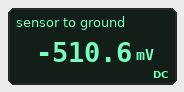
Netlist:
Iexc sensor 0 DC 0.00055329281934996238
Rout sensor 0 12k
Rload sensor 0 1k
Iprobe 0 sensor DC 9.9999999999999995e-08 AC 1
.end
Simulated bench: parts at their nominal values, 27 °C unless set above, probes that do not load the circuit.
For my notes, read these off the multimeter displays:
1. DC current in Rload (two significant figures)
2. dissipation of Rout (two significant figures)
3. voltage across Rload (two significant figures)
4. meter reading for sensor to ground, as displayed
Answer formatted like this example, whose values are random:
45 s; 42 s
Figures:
510 µA; 22 µW; 510 mV; -510.6 mV
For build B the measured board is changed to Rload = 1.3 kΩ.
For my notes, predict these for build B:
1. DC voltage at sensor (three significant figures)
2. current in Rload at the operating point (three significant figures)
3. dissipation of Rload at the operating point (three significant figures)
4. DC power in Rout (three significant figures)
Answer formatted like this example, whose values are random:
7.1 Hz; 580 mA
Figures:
-649 mV; 499 µA; 324 µW; 35.1 µW
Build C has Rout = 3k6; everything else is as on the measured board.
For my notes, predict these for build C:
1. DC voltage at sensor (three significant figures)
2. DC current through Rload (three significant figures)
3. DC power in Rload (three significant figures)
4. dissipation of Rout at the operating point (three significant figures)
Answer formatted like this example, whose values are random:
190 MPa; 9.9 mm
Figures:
-433 mV; 433 µA; 187 µW; 52.1 µW
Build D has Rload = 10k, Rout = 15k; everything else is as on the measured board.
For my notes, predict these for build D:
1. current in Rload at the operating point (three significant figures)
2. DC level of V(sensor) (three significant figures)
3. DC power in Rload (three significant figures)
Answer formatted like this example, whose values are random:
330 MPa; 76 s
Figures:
332 µA; -3.32 V; 1.10 mW
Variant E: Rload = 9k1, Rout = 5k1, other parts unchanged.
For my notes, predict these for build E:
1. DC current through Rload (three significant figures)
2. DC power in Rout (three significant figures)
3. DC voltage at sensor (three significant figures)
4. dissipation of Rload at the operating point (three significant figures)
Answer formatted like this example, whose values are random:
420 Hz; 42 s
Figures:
199 µA; 641 µW; -1.81 V; 359 µW
